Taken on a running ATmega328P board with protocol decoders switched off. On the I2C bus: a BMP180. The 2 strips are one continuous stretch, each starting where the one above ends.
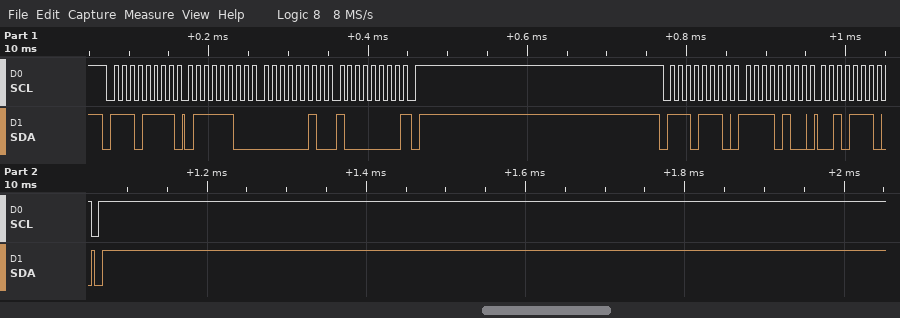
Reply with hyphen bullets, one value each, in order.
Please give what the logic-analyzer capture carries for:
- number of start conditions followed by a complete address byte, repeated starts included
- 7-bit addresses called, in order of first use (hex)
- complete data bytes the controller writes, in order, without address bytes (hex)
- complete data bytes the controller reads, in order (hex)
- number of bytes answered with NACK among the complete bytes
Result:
- 2
- 0x77
- F4 2E
- 7C 02 80
- 1
